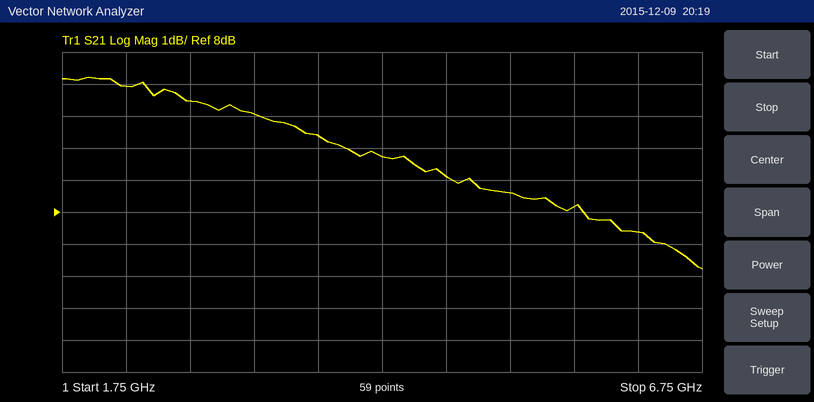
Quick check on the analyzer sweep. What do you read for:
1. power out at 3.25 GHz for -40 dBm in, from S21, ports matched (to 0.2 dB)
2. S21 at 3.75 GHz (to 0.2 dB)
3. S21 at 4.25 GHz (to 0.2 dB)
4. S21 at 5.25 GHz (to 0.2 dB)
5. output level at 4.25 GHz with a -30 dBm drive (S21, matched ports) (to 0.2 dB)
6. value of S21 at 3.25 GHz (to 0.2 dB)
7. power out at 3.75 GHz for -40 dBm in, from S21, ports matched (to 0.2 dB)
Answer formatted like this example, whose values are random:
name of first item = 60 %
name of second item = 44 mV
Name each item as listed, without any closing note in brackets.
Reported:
power out at 3.25 GHz for -40 dBm in, from S21, ports matched = -29.0 dBm
S21 at 3.75 GHz = 10.4 dB
S21 at 4.25 GHz = 9.8 dB
S21 at 5.25 GHz = 8.6 dB
output level at 4.25 GHz with a -30 dBm drive (S21, matched ports) = -20.2 dBm
value of S21 at 3.25 GHz = 11.0 dB
power out at 3.75 GHz for -40 dBm in, from S21, ports matched = -29.6 dBm
